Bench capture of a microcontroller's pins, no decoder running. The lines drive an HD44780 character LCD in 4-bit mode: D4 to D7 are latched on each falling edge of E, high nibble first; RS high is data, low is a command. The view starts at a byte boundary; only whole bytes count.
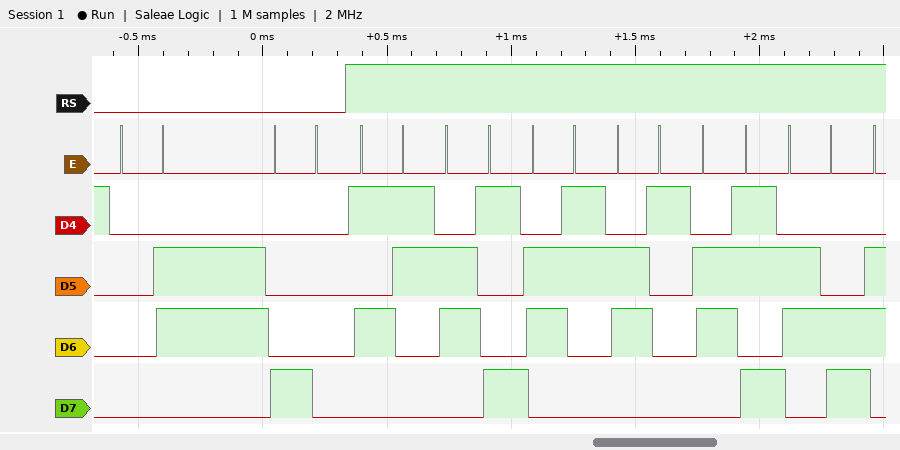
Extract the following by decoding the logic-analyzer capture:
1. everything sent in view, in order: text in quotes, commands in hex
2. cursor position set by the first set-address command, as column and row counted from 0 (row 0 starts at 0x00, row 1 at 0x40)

0x06 0x80 "Sicakl"
column 0, row 0
